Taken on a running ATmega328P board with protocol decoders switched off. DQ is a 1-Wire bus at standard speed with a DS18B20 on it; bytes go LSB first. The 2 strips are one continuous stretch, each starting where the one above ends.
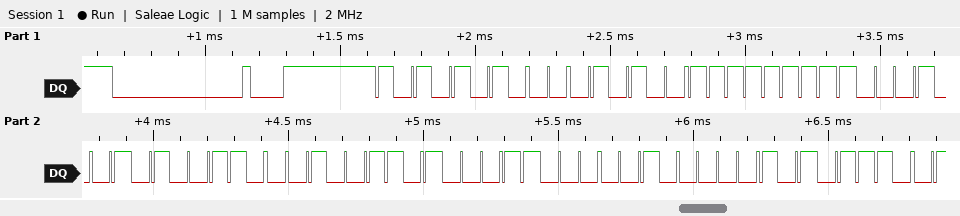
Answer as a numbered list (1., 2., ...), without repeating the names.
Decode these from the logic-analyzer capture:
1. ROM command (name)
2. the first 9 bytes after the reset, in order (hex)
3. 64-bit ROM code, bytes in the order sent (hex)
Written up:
1. Match ROM
2. 55 28 FF 91 32 B2 18 04 75
3. 28 FF 91 32 B2 18 04 75
